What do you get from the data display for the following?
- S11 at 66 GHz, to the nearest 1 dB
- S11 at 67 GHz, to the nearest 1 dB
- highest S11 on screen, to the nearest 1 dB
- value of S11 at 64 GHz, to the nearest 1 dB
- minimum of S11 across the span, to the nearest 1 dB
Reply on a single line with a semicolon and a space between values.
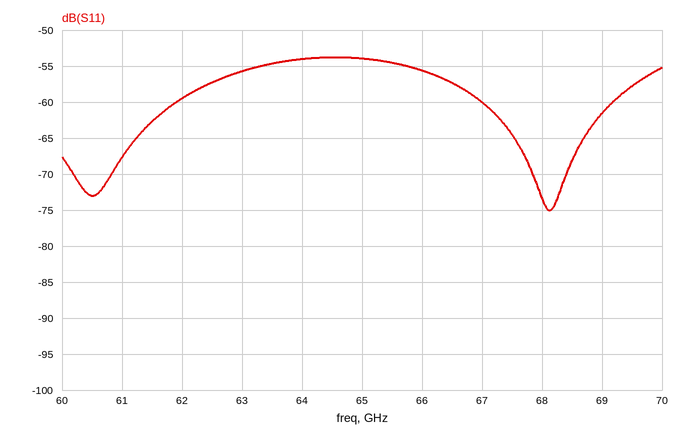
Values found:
-56 dB; -60 dB; -54 dB; -54 dB; -75 dB
